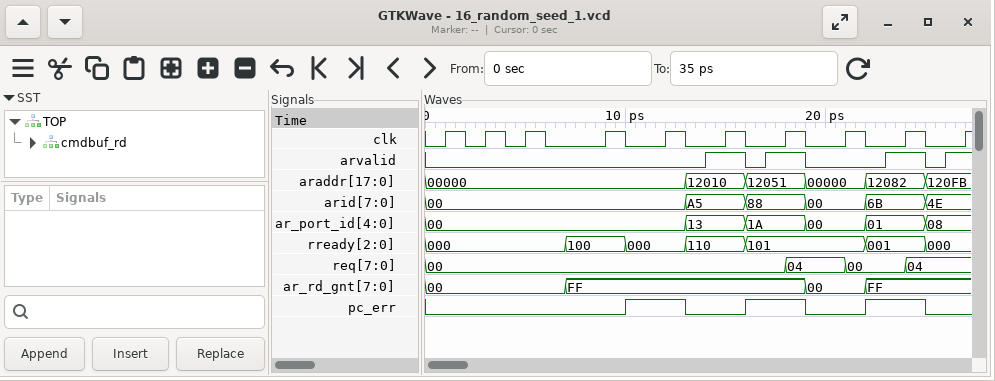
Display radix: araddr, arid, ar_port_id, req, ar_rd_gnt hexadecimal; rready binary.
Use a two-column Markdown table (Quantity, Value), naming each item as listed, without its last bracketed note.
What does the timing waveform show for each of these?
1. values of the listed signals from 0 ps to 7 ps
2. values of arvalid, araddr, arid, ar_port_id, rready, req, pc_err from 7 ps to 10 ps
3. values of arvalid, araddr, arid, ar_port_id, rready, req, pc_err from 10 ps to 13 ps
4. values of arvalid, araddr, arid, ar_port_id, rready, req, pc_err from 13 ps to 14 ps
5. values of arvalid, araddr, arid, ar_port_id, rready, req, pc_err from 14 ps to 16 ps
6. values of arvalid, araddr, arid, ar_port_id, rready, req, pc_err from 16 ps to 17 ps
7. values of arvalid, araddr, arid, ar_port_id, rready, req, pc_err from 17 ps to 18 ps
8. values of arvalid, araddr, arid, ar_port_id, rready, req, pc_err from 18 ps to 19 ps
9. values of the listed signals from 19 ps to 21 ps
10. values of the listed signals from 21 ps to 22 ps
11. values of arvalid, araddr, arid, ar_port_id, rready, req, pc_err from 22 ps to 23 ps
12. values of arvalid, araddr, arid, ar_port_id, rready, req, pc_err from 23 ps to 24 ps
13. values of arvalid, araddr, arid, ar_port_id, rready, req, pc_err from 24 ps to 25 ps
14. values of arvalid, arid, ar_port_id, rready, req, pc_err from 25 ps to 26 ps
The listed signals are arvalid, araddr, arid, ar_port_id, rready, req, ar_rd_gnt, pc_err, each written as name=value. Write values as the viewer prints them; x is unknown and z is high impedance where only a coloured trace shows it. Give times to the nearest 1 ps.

| Quantity | Value |
|---|---|
| values of the listed signals from 0 ps to 7 ps | arvalid=0, araddr=00000, arid=00, ar_port_id=00, rready=000, req=00, ar_rd_gnt=00, pc_err=0 |
| values of arvalid, araddr, arid, ar_port_id, rready, req, pc_err from 7 ps to 10 ps | arvalid=0, araddr=00000, arid=00, ar_port_id=00, rready=100, req=00, pc_err=0 |
| values of arvalid, araddr, arid, ar_port_id, rready, req, pc_err from 10 ps to 13 ps | arvalid=0, araddr=00000, arid=00, ar_port_id=00, rready=000, req=00, pc_err=1 |
| values of arvalid, araddr, arid, ar_port_id, rready, req, pc_err from 13 ps to 14 ps | arvalid=0, araddr=12010, arid=A5, ar_port_id=13, rready=110, req=00, pc_err=0 |
| values of arvalid, araddr, arid, ar_port_id, rready, req, pc_err from 14 ps to 16 ps | arvalid=1, araddr=12010, arid=A5, ar_port_id=13, rready=110, req=00, pc_err=0 |
| values of arvalid, araddr, arid, ar_port_id, rready, req, pc_err from 16 ps to 17 ps | arvalid=0, araddr=12051, arid=88, ar_port_id=1A, rready=101, req=00, pc_err=1 |
| values of arvalid, araddr, arid, ar_port_id, rready, req, pc_err from 17 ps to 18 ps | arvalid=1, araddr=12051, arid=88, ar_port_id=1A, rready=101, req=00, pc_err=1 |
| values of arvalid, araddr, arid, ar_port_id, rready, req, pc_err from 18 ps to 19 ps | arvalid=1, araddr=12051, arid=88, ar_port_id=1A, rready=101, req=04, pc_err=1 |
| values of the listed signals from 19 ps to 21 ps | arvalid=0, araddr=00000, arid=00, ar_port_id=00, rready=101, req=04, ar_rd_gnt=00, pc_err=0 |
| values of the listed signals from 21 ps to 22 ps | arvalid=0, araddr=00000, arid=00, ar_port_id=00, rready=101, req=00, ar_rd_gnt=00, pc_err=0 |
| values of arvalid, araddr, arid, ar_port_id, rready, req, pc_err from 22 ps to 23 ps | arvalid=0, araddr=12082, arid=6B, ar_port_id=01, rready=001, req=00, pc_err=1 |
| values of arvalid, araddr, arid, ar_port_id, rready, req, pc_err from 23 ps to 24 ps | arvalid=1, araddr=12082, arid=6B, ar_port_id=01, rready=001, req=00, pc_err=1 |
| values of arvalid, araddr, arid, ar_port_id, rready, req, pc_err from 24 ps to 25 ps | arvalid=1, araddr=12082, arid=6B, ar_port_id=01, rready=001, req=04, pc_err=1 |
| values of arvalid, arid, ar_port_id, rready, req, pc_err from 25 ps to 26 ps | arvalid=0, arid=4E, ar_port_id=08, rready=000, req=04, pc_err=0 |
